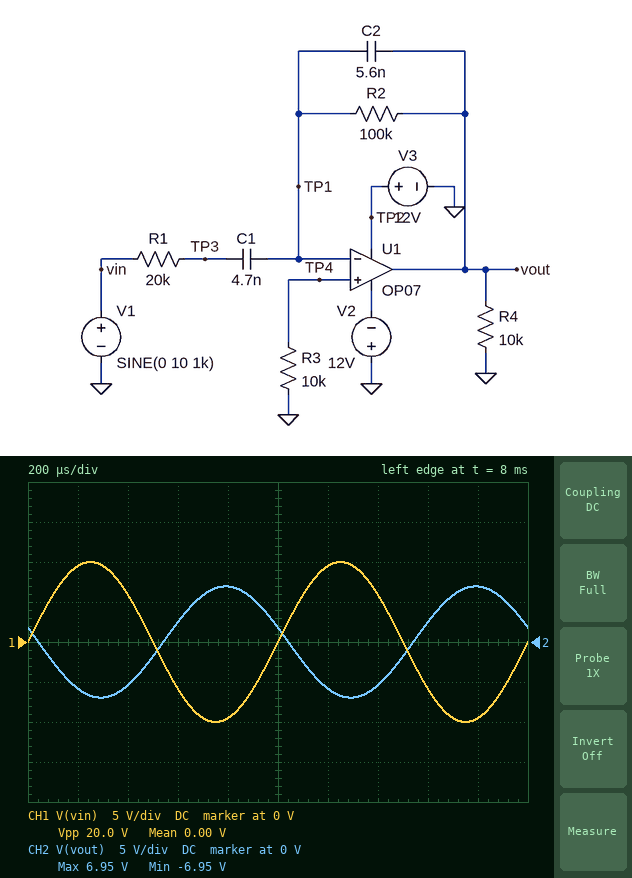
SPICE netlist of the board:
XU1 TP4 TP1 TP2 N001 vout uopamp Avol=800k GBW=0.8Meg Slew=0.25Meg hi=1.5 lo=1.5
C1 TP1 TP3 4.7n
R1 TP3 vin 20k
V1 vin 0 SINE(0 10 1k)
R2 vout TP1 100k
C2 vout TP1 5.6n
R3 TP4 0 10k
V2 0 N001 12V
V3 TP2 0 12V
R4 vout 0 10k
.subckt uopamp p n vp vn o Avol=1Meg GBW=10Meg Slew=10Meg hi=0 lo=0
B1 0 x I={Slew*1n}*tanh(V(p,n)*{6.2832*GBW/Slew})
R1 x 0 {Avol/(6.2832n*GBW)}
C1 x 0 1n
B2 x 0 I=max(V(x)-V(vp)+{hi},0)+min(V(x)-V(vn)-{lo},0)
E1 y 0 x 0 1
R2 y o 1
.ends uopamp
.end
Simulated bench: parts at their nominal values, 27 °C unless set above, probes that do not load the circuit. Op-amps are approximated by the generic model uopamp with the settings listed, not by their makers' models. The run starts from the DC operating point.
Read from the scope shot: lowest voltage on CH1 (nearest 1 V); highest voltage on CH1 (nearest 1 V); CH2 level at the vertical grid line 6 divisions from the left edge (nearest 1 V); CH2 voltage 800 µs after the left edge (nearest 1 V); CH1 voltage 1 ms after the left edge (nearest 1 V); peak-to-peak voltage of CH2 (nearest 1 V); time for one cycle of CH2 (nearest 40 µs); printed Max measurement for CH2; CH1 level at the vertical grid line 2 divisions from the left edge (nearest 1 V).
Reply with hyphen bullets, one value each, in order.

- -10 V
- 10 V
- -6 V
- 7 V
- 0 V
- 14 V
- 1.00 ms
- 6.95 V
- 6 V
